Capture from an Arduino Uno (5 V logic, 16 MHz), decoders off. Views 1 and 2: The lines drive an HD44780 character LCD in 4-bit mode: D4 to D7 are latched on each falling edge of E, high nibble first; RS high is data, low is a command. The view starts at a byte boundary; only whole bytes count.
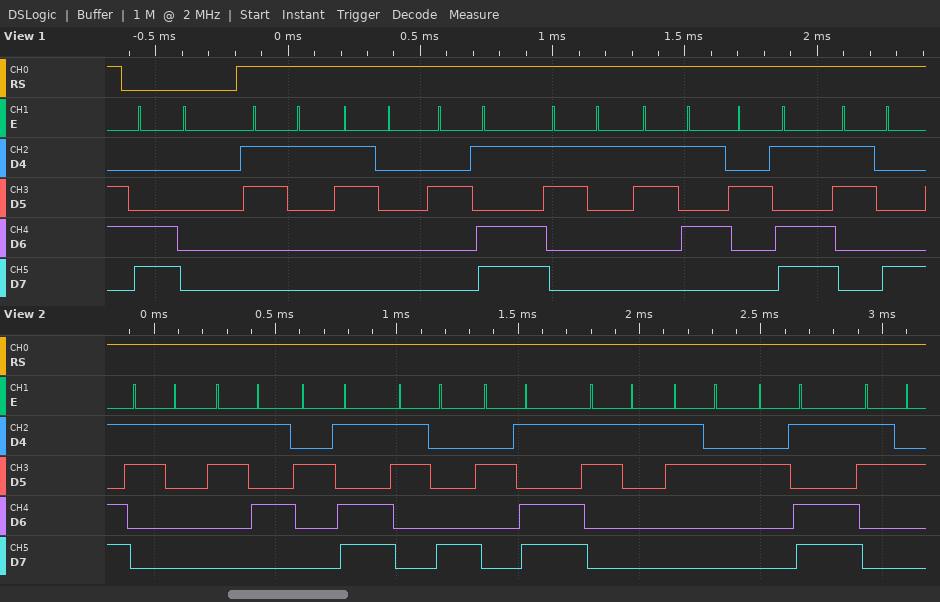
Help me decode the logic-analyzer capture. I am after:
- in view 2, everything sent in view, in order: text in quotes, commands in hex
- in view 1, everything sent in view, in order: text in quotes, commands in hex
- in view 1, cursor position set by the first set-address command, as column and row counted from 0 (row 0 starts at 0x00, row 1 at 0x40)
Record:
"15-8-12-2"
0xC0 "10-15-8"
column 0, row 1
